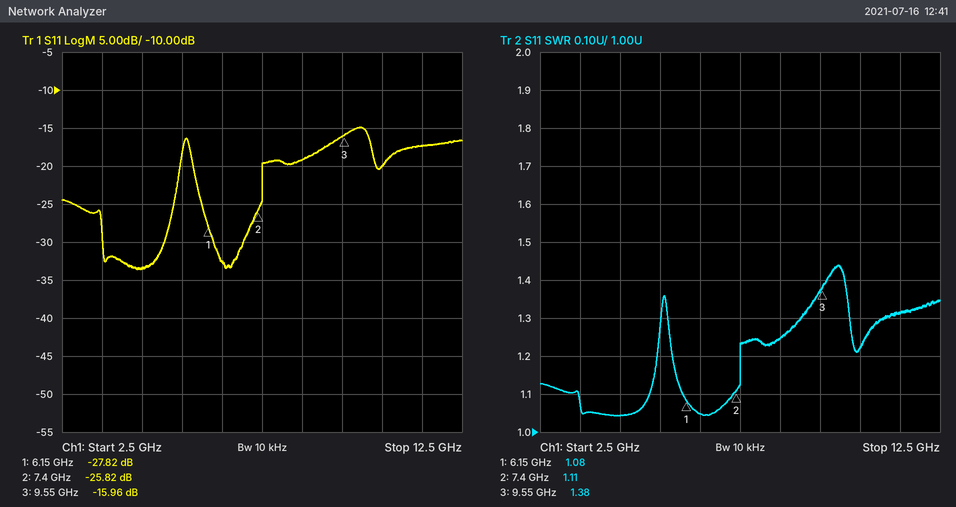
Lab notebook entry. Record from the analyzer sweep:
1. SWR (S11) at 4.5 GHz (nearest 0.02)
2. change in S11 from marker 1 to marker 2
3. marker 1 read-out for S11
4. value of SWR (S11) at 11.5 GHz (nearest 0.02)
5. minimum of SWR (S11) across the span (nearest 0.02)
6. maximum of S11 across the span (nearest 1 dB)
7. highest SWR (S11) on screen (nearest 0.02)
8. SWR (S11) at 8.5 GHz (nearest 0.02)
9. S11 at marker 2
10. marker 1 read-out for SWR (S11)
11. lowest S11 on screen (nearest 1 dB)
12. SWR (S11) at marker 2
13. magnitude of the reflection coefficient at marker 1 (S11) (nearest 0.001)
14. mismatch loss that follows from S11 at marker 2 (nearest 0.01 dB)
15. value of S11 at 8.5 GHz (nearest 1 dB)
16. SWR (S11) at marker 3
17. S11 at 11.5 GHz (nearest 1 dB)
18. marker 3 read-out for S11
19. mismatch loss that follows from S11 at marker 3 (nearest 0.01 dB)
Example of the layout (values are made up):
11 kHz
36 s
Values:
1.04
2.00 dB
-27.82 dB
1.32
1.04
-15 dB
1.44
1.24
-25.82 dB
1.08
-34 dB
1.11
0.041
0.01 dB
-19 dB
1.38
-17 dB
-15.96 dB
0.11 dB
